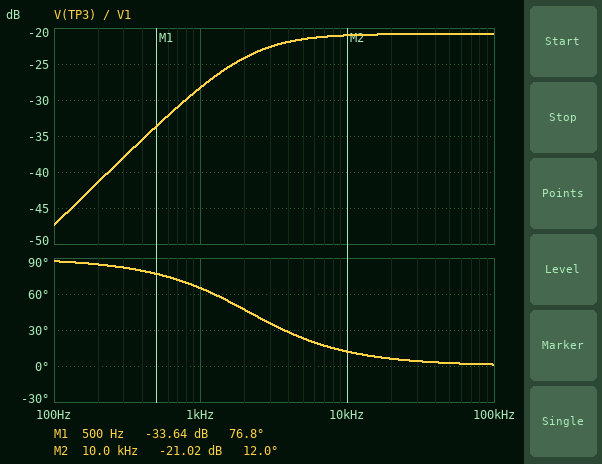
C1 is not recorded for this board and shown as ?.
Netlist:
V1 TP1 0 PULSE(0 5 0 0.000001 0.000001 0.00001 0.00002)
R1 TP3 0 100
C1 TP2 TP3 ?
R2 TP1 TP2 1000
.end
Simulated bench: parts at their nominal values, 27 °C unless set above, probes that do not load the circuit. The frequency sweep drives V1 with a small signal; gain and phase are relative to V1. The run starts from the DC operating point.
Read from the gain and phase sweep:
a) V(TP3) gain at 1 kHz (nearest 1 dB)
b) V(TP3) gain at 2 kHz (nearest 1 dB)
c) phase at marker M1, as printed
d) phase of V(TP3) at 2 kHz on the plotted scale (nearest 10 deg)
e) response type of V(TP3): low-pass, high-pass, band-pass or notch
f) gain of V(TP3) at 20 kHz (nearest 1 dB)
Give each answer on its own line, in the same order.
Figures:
-28 dB
-24 dB
76.8 deg
50 deg
high-pass
-21 dB
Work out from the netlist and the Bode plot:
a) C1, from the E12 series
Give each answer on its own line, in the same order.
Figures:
68 nF
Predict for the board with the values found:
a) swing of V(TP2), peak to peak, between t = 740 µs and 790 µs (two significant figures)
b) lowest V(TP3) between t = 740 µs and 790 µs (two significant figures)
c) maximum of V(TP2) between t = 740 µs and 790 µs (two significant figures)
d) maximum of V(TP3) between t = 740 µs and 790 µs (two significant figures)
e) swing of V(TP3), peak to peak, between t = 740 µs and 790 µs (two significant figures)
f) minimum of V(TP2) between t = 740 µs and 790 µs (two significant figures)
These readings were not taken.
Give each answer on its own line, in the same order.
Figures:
730 mV
-260 mV
3.1 V
220 mV
480 mV
2.4 V
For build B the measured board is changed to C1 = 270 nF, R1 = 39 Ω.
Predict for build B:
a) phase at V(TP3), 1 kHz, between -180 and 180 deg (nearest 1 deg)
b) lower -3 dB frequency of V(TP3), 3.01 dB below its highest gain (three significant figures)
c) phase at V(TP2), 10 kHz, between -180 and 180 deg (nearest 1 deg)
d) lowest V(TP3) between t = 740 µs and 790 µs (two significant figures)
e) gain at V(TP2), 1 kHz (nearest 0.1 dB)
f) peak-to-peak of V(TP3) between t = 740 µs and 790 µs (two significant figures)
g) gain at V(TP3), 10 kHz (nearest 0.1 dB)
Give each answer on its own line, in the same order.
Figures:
30 deg
567 Hz
-53 deg
-98 mV
-6.1 dB
190 mV
-28.5 dB
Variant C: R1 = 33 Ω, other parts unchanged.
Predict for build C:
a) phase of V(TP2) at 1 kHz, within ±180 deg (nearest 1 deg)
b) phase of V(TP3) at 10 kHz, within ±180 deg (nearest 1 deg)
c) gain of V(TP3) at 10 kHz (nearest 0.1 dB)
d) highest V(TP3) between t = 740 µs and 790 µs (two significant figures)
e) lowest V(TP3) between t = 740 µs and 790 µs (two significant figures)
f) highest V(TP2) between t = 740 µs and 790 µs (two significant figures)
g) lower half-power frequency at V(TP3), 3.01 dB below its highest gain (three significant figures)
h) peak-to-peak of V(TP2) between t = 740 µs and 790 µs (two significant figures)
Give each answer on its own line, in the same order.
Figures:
-23 deg
13 deg
-30.1 dB
77 mV
-93 mV
3.0 V
2.27 kHz
470 mV
